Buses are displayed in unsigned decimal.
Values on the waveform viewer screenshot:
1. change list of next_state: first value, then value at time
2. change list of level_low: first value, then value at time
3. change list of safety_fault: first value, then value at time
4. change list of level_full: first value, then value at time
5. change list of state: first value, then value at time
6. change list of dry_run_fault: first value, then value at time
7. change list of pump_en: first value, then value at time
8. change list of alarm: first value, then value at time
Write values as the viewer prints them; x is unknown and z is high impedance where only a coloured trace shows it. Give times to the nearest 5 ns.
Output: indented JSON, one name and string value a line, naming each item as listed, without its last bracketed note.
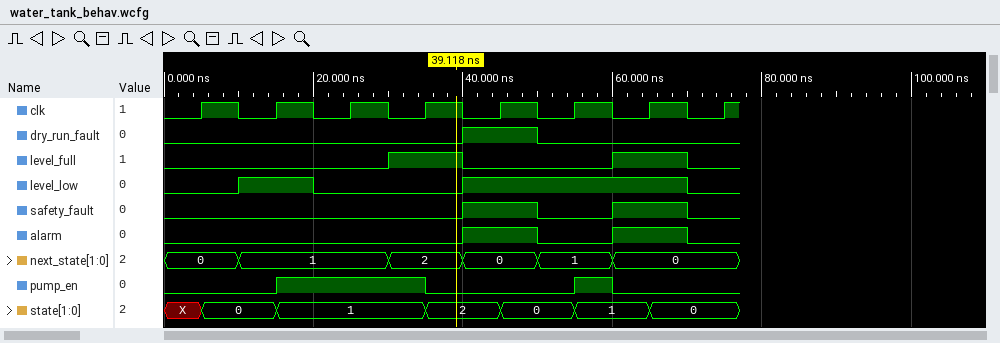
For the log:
{
  "change list of next_state: first value, then value at time": "0, 1 at 10 ns, 2 at 30 ns, 0 at 40 ns, 1 at 50 ns, 0 at 60 ns",
  "change list of level_low: first value, then value at time": "0, 1 at 10 ns, 0 at 20 ns, 1 at 40 ns, 0 at 70 ns",
  "change list of safety_fault: first value, then value at time": "0, 1 at 40 ns, 0 at 50 ns, 1 at 60 ns, 0 at 70 ns",
  "change list of level_full: first value, then value at time": "0, 1 at 30 ns, 0 at 40 ns, 1 at 60 ns, 0 at 70 ns",
  "change list of state: first value, then value at time": "X, 0 at 5 ns, 1 at 15 ns, 2 at 35 ns, 0 at 45 ns, 1 at 55 ns, 0 at 65 ns",
  "change list of dry_run_fault: first value, then value at time": "0, 1 at 40 ns, 0 at 50 ns",
  "change list of pump_en: first value, then value at time": "0, 1 at 15 ns, 0 at 35 ns, 1 at 55 ns, 0 at 60 ns",
  "change list of alarm: first value, then value at time": "0, 1 at 40 ns, 0 at 50 ns, 1 at 60 ns, 0 at 70 ns"
}
